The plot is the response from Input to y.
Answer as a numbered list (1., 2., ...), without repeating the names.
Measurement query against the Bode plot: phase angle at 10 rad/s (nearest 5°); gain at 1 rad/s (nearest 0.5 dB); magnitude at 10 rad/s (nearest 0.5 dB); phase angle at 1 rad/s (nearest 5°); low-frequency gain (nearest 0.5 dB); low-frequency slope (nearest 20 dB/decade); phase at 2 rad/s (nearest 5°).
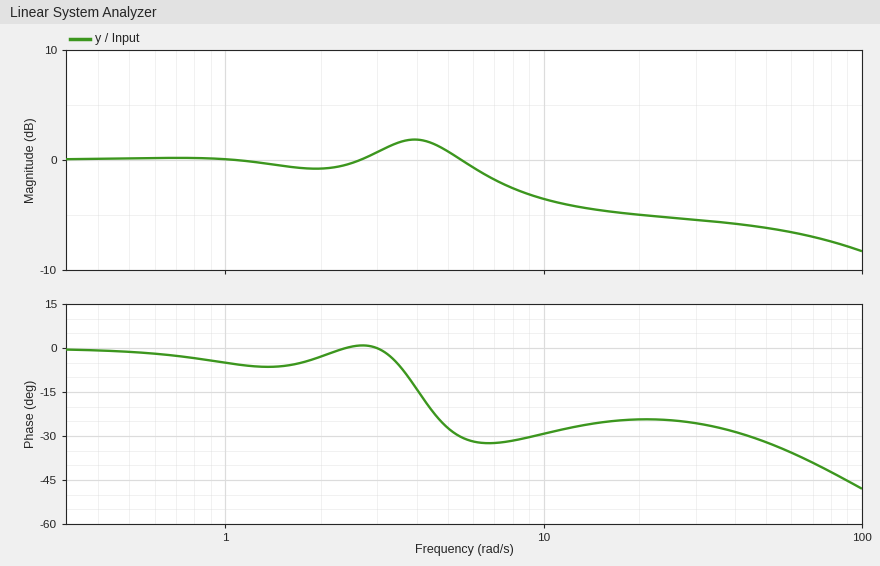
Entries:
1. -30°
2. 0.0 dB
3. -3.5 dB
4. -5°
5. 0.0 dB
6. 0 dB/decade
7. -5°
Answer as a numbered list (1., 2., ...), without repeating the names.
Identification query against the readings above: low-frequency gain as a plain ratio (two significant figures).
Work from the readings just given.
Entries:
1. 1.0
